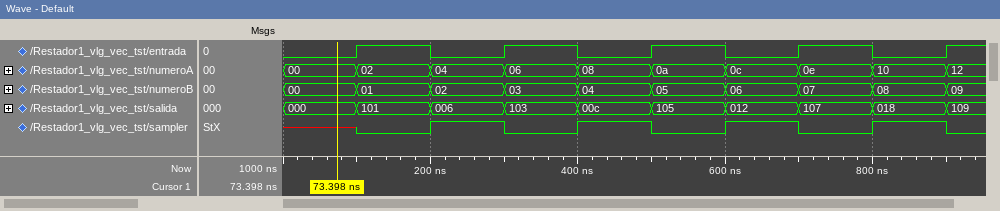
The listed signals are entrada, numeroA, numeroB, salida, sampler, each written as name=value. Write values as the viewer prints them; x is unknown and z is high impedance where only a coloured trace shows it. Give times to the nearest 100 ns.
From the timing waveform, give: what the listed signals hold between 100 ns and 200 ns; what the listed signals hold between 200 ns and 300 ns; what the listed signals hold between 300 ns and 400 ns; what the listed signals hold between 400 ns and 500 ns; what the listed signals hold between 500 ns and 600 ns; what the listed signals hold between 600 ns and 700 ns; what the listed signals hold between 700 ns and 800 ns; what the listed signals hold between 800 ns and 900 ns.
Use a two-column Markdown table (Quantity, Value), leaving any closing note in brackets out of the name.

| Quantity | Value |
|---|---|
| what the listed signals hold between 100 ns and 200 ns | entrada=1, numeroA=02, numeroB=01, salida=101, sampler=0 |
| what the listed signals hold between 200 ns and 300 ns | entrada=0, numeroA=04, numeroB=02, salida=006, sampler=1 |
| what the listed signals hold between 300 ns and 400 ns | entrada=1, numeroA=06, numeroB=03, salida=103, sampler=0 |
| what the listed signals hold between 400 ns and 500 ns | entrada=0, numeroA=08, numeroB=04, salida=00c, sampler=1 |
| what the listed signals hold between 500 ns and 600 ns | entrada=1, numeroA=0a, numeroB=05, salida=105, sampler=0 |
| what the listed signals hold between 600 ns and 700 ns | entrada=0, numeroA=0c, numeroB=06, salida=012, sampler=1 |
| what the listed signals hold between 700 ns and 800 ns | entrada=1, numeroA=0e, numeroB=07, salida=107, sampler=0 |
| what the listed signals hold between 800 ns and 900 ns | entrada=0, numeroA=10, numeroB=08, salida=018, sampler=1 |
